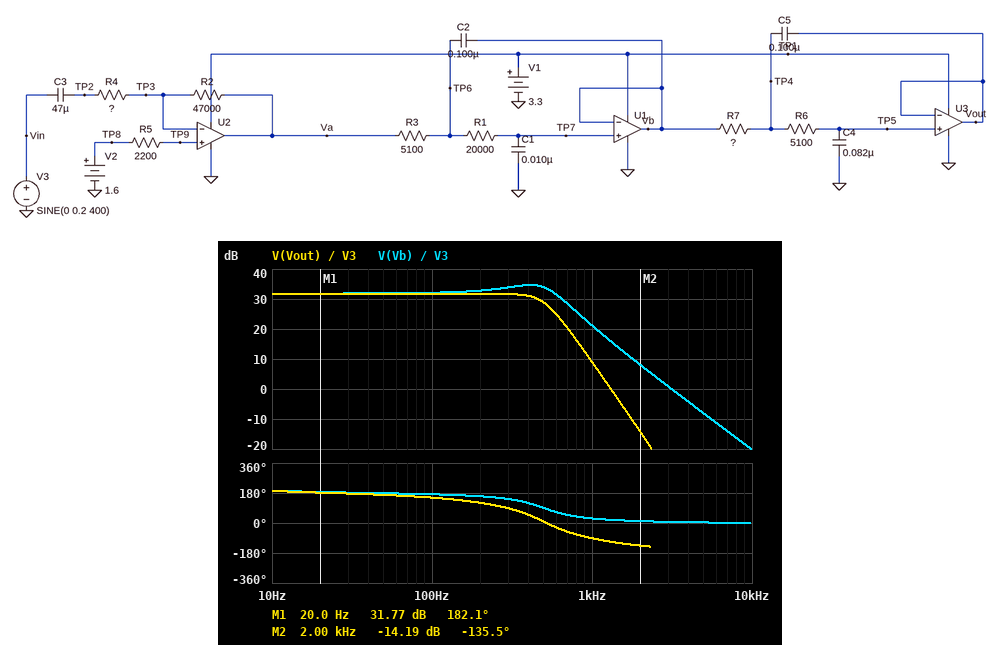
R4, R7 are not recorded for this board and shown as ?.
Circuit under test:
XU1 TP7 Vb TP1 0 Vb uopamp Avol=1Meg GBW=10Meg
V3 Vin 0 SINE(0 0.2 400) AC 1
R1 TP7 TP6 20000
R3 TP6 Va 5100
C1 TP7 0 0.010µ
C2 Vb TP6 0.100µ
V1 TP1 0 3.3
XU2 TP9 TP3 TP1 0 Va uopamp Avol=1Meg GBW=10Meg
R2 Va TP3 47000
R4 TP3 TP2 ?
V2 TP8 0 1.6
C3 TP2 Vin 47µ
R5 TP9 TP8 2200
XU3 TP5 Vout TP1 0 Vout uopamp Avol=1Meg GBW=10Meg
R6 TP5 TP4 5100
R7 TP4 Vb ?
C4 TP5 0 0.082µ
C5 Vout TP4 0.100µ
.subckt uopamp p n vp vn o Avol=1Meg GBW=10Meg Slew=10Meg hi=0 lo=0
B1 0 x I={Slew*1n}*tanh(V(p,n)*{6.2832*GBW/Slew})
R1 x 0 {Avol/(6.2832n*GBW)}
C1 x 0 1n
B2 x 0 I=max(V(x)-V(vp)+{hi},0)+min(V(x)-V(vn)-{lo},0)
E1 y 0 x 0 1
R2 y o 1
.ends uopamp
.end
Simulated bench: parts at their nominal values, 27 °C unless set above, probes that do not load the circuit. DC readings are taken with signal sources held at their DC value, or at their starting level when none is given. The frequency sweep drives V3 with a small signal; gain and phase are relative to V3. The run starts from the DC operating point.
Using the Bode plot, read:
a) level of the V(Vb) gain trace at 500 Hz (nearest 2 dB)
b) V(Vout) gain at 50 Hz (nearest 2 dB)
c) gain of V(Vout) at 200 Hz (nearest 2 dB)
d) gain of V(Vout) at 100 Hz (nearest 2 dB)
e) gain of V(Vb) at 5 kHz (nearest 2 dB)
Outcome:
34 dB
32 dB
32 dB
32 dB
-8 dB
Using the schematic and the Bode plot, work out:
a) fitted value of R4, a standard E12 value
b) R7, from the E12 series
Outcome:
1.2 kΩ
1.8 kΩ
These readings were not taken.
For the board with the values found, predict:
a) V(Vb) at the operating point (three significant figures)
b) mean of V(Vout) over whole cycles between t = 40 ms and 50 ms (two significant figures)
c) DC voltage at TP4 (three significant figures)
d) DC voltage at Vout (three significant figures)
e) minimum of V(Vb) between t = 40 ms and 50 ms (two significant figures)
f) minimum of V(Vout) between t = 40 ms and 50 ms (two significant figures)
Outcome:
1.60 V
1.6 V
1.60 V
1.60 V
-9.9 mV
350 mV
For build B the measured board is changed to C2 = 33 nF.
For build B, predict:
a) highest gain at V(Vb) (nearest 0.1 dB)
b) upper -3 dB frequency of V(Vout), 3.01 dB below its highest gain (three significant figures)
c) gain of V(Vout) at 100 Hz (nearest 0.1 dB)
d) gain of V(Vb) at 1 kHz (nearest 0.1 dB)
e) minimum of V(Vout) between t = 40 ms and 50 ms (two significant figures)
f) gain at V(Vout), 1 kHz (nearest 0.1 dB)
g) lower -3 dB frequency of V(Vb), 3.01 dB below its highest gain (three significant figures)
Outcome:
31.9 dB
360 Hz
31.6 dB
27.7 dB
330 mV
15.5 dB
2.83 Hz
